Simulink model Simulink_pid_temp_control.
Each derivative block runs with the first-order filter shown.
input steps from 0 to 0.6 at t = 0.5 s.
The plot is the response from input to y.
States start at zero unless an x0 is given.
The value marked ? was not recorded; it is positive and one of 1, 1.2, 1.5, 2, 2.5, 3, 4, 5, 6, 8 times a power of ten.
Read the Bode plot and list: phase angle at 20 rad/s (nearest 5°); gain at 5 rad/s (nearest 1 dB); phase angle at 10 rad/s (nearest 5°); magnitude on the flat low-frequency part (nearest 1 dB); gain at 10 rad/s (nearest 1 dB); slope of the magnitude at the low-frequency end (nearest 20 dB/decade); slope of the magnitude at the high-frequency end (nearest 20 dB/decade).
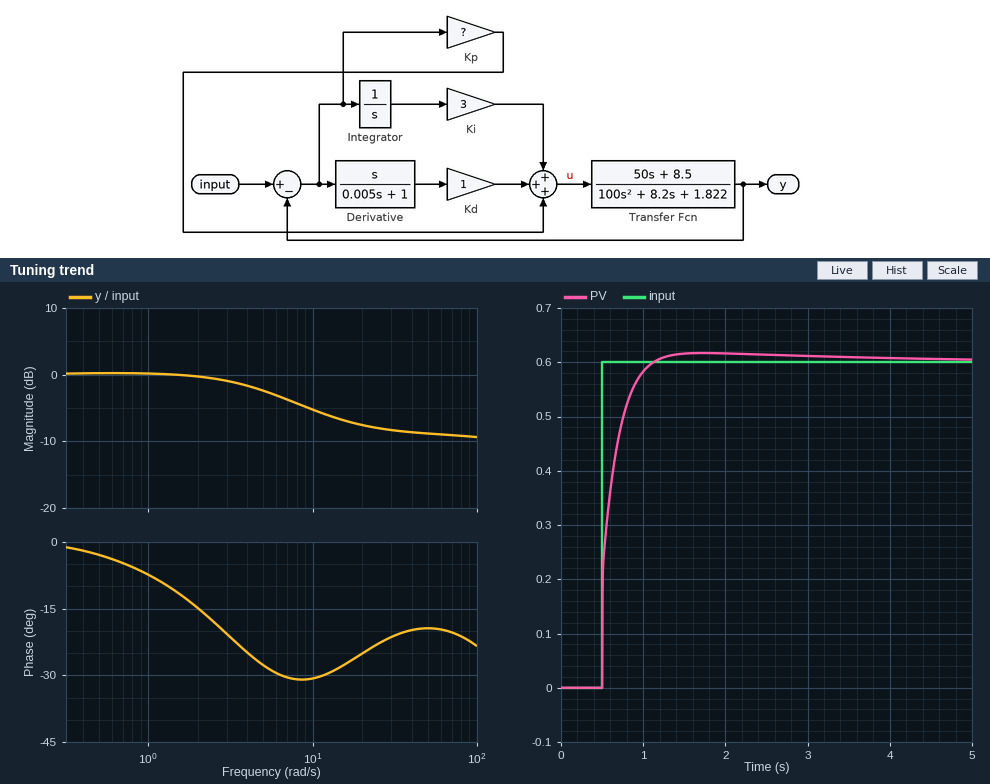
-25°
-2 dB
-30°
0 dB
-5 dB
0 dB/decade
0 dB/decade
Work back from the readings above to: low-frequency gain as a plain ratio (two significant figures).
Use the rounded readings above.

1.0
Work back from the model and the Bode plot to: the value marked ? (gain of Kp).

15
